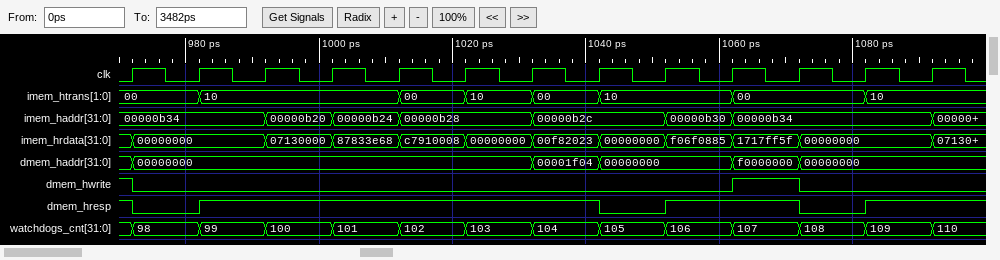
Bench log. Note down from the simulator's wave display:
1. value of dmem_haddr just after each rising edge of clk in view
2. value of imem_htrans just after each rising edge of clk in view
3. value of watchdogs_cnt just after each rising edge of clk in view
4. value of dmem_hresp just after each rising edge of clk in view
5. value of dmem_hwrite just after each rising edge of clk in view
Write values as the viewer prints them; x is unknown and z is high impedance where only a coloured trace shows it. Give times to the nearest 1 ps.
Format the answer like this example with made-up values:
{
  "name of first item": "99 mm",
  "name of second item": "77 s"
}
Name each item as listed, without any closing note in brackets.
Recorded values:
{
  "value of dmem_haddr just after each rising edge of clk in view": "00000000, 00000000, 00000000, 00000000, 00000000, 00000000, 00001f04, 00000000, 00000000, f0000000, 00000000, 00000000, 00000000",
  "value of imem_htrans just after each rising edge of clk in view": "00, 10, 10, 10, 00, 10, 00, 10, 10, 00, 00, 10, 10",
  "value of watchdogs_cnt just after each rising edge of clk in view": "98, 99, 100, 101, 102, 103, 104, 105, 106, 107, 108, 109, 110",
  "value of dmem_hresp just after each rising edge of clk in view": "0 1 1 1 1 1 1 0 1 1 0 1 1",
  "value of dmem_hwrite just after each rising edge of clk in view": "0 0 0 0 0 0 0 0 0 1 0 0 0"
}
